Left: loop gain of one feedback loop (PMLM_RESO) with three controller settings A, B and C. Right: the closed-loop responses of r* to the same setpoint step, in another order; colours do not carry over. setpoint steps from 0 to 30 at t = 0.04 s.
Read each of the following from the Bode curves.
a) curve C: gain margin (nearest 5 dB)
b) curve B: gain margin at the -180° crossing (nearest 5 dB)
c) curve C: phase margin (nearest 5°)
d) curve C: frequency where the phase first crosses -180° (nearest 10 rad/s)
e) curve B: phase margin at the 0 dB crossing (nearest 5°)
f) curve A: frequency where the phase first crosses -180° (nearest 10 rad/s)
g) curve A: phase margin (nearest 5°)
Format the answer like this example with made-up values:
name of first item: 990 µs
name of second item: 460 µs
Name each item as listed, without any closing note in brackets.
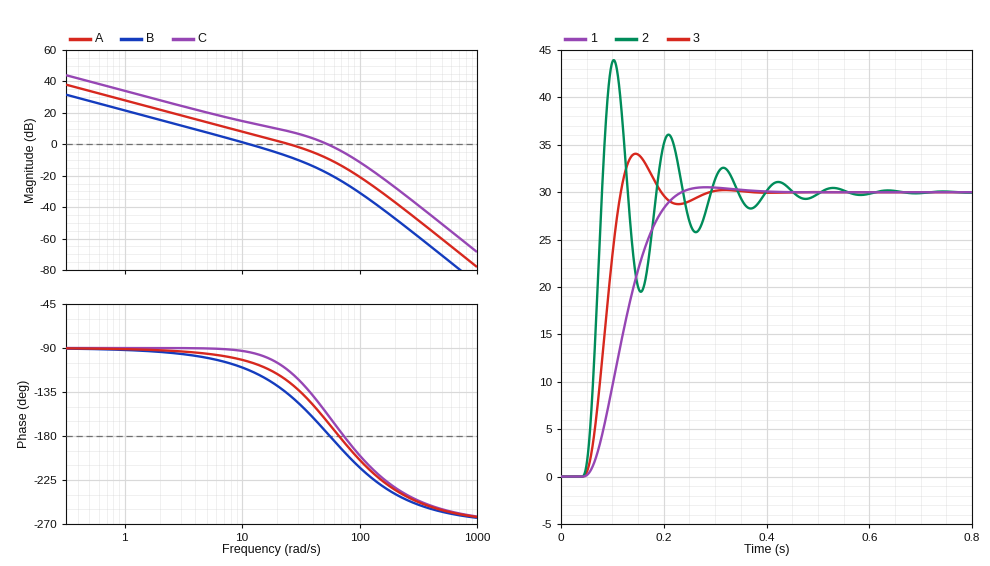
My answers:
curve C: gain margin: 5 dB
curve B: gain margin at the -180° crossing: 20 dB
curve C: phase margin: 20°
curve C: frequency where the phase first crosses -180°: 70 rad/s
curve B: phase margin at the 0 dB crossing: 65°
curve A: frequency where the phase first crosses -180°: 70 rad/s
curve A: phase margin: 55°
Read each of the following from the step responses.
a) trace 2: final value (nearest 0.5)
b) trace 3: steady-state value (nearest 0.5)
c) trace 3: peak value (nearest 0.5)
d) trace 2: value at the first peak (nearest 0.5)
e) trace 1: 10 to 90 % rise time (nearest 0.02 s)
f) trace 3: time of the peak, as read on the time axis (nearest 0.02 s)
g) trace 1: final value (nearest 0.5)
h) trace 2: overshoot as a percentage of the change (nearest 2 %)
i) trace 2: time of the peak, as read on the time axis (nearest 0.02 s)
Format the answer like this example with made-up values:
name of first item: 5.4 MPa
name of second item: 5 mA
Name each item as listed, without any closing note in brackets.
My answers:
trace 2: final value: 30.0
trace 3: steady-state value: 30.0
trace 3: peak value: 34.0
trace 2: value at the first peak: 44.0
trace 1: 10 to 90 % rise time: 0.12 s
trace 3: time of the peak, as read on the time axis: 0.14 s
trace 1: final value: 30.0
trace 2: overshoot as a percentage of the change: 46 %
trace 2: time of the peak, as read on the time axis: 0.10 s
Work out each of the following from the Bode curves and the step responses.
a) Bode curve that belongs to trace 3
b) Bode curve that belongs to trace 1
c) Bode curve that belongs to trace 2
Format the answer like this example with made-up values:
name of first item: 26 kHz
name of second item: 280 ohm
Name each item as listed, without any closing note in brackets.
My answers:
Bode curve that belongs to trace 3: A
Bode curve that belongs to trace 1: B
Bode curve that belongs to trace 2: C
